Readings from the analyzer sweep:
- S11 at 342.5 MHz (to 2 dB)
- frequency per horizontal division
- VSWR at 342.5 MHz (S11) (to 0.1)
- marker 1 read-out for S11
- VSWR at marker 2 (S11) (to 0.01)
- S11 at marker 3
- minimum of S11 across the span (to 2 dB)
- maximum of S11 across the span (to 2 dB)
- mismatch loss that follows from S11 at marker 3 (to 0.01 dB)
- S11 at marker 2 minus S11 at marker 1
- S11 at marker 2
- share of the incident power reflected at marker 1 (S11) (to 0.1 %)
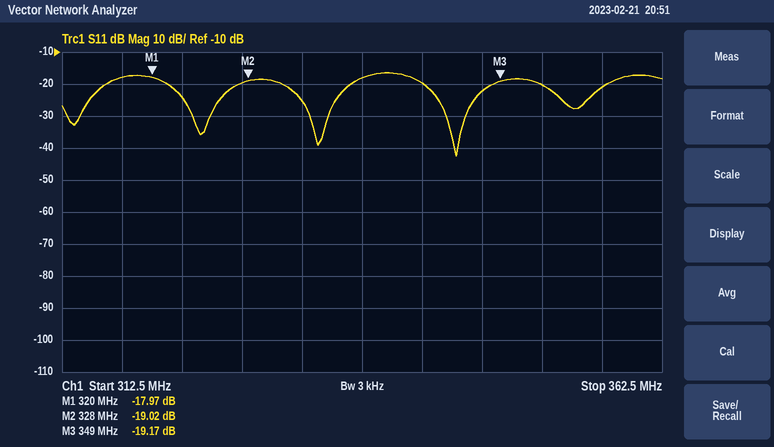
-20 dB
5 MHz
1.2
-17.97 dB
1.25
-19.17 dB
-42 dB
-16 dB
0.05 dB
-1.05 dB
-19.02 dB
1.6 %
